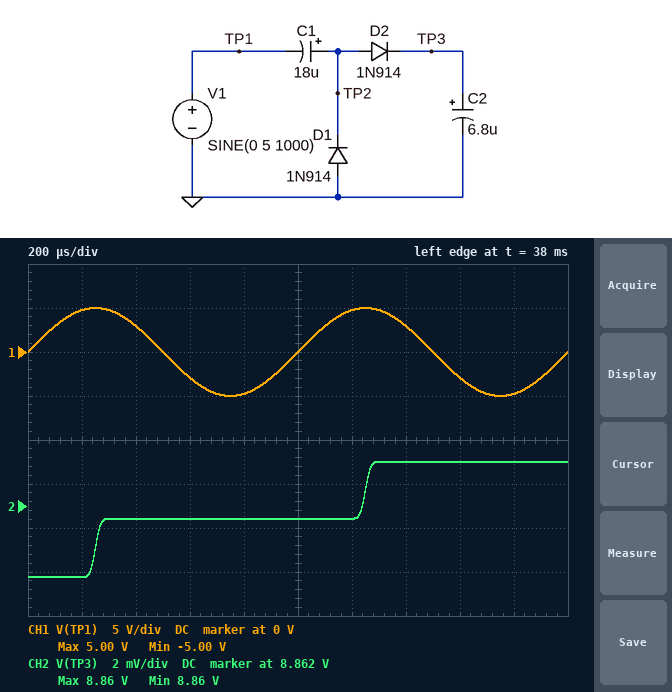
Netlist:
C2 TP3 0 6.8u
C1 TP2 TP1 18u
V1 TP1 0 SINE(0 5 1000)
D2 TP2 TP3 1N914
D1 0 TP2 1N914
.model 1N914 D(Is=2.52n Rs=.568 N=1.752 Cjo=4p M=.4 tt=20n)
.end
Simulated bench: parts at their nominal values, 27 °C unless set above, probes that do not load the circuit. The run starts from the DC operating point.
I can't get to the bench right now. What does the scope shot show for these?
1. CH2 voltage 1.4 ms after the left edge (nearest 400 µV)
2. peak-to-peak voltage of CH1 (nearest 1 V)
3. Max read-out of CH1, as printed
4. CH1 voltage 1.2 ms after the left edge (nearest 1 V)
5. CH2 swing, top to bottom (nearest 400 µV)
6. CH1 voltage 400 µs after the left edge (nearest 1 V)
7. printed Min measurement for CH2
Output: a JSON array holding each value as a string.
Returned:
["8.8640 V", "10 V", "5.00 V", "5 V", "5.2 mV", "3 V", "8.86 V"]
